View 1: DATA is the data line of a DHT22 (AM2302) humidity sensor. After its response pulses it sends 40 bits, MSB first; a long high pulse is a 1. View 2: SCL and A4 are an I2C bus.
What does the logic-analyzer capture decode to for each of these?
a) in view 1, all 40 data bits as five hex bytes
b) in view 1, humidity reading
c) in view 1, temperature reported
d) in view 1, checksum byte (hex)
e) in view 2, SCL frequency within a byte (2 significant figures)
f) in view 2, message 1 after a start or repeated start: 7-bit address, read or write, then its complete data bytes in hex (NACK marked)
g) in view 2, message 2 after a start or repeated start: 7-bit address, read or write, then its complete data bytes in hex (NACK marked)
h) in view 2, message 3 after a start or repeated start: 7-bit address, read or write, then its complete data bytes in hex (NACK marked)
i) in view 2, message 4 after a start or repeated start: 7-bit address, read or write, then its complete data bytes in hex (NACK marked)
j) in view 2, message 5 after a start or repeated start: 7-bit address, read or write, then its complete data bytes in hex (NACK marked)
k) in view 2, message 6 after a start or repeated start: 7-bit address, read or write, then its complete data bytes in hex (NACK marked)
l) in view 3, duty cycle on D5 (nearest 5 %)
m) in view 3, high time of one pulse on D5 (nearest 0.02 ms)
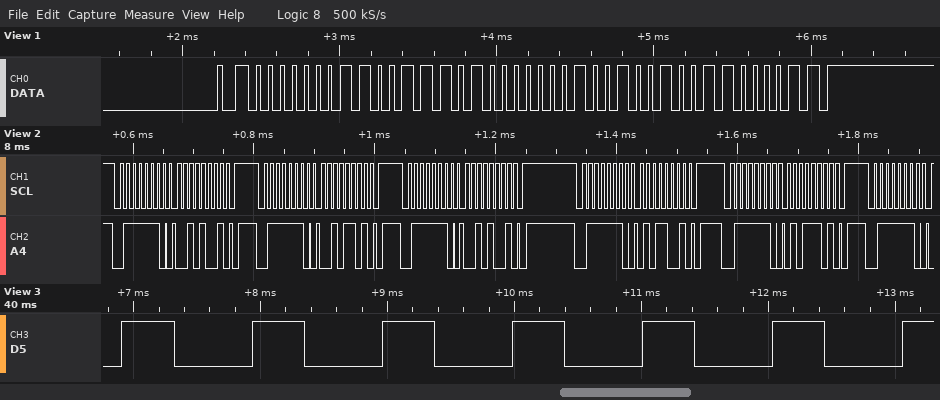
01 9D 01 24 C3
41.3 %
29.2 °C
0xC3
100 kHz
0x3F write: 29
0x3F write: 2D
0x3F write: 29
0x3F write: 59
0x3F write: 5D
0x3F write
40 %
0.42 ms
